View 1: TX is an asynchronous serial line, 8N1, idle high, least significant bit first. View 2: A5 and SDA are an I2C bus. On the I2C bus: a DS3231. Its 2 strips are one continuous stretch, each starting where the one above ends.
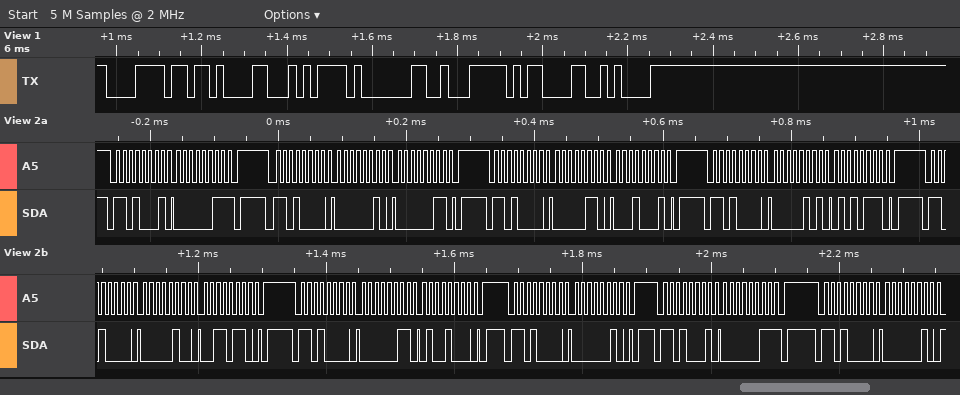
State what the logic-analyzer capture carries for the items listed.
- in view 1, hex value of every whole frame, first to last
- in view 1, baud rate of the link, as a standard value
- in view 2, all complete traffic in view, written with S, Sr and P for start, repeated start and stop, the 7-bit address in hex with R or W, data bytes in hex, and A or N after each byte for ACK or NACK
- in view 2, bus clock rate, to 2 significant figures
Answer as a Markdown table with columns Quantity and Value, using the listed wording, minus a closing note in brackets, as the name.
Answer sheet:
| Quantity | Value |
|---|---|
| in view 1, hex value of every whole frame, first to last | 78 0B D4 01 E2 0D 0A |
| in view 1, baud rate of the link, as a standard value | 57600 baud |
| in view 2, all complete traffic in view, written with S, Sr and P for start, repeated start and stop, the 7-bit address in hex with R or W, data bytes in hex, and A or N after each byte for ACK or NACK | S 68R A 03 N P S 68W A 02 A 03 A P S 68W A 06 A 11 A P S 68W A 05 A 57 A P S 68W A 04 A 36 A P S 68W A 03 A 48 A P S 68W A 02 A P S 68R A 03 N P S 68W A 02 A |
| in view 2, bus clock rate, to 2 significant figures | 100 kHz |
